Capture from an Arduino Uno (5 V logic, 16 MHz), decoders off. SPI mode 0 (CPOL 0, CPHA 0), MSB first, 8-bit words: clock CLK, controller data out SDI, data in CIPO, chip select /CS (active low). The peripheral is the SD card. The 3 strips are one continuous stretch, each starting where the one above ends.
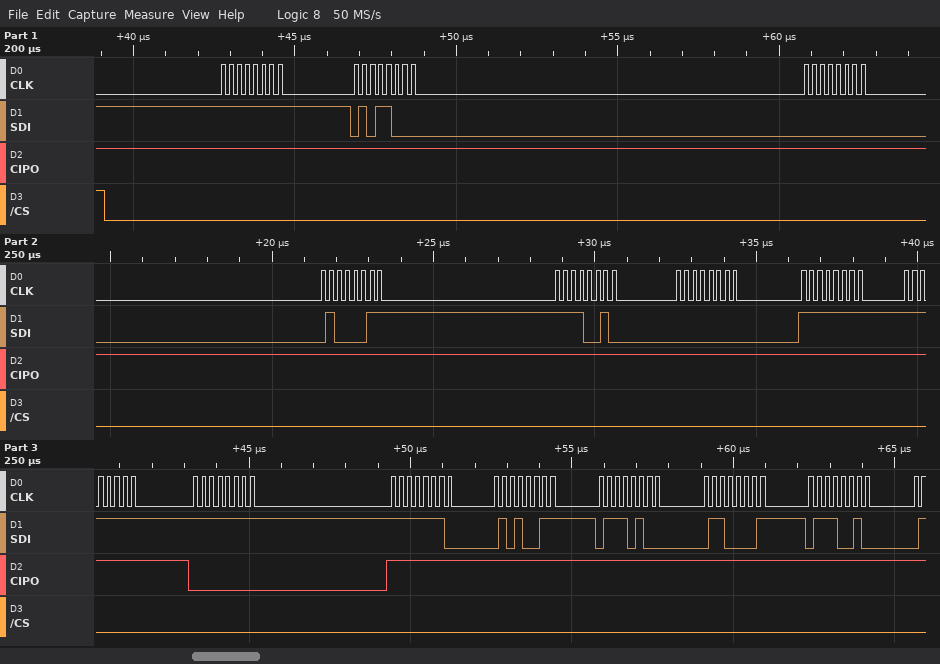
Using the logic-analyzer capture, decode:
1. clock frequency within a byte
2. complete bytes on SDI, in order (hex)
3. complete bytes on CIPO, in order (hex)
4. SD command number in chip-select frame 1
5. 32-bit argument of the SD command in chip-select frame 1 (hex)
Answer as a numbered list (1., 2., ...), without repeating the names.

1. 4 MHz
2. FF 58 00 43 F2 00 FF FF FF FE 53 74 61 72
3. FF FF FF FF FF FF FF FF 00 FF FF FF FF FF
4. CMD24
5. 0x0043F200
